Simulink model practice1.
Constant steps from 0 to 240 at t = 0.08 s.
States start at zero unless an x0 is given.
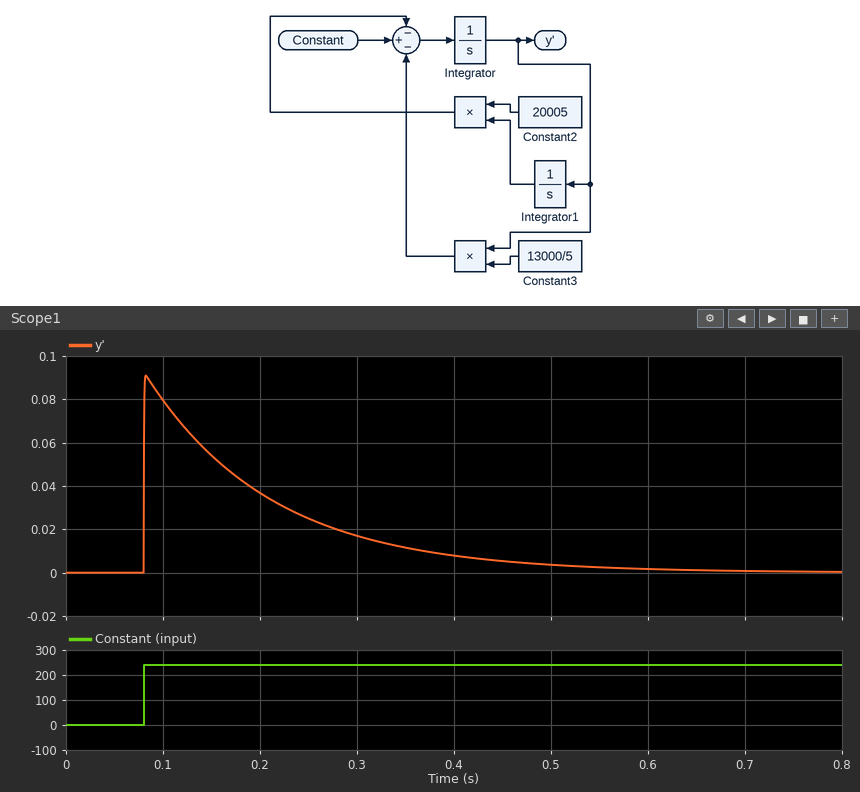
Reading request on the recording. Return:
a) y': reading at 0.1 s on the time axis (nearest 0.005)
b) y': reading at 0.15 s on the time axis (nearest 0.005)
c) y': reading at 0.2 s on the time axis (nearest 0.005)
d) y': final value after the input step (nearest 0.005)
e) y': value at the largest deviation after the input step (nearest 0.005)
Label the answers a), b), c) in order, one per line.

a) 0.080
b) 0.055
c) 0.035
d) 0.000
e) 0.090
